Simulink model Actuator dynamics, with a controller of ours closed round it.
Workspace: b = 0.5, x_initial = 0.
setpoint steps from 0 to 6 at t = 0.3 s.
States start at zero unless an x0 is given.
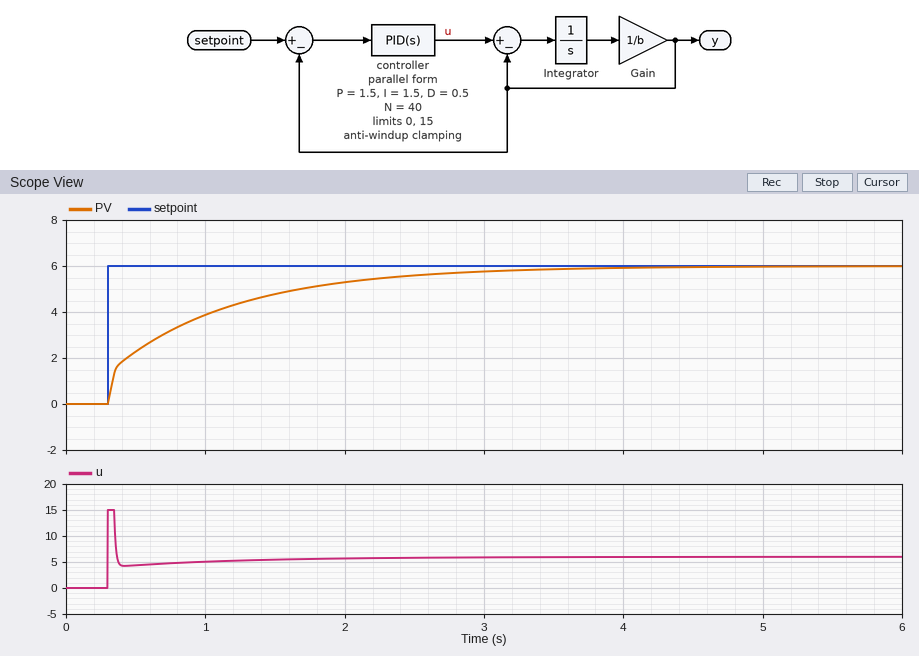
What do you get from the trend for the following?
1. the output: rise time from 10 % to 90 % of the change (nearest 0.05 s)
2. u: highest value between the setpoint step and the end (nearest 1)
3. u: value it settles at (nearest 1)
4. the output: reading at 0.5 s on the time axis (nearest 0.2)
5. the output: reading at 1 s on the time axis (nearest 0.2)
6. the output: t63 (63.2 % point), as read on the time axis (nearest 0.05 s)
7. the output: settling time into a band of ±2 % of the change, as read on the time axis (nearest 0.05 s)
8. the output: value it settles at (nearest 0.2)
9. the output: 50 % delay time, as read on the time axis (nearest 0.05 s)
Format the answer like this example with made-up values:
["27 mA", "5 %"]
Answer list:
["1.85 s", "15", "6", "2.2", "3.8", "0.95 s", "3.65 s", "6.0", "0.70 s"]
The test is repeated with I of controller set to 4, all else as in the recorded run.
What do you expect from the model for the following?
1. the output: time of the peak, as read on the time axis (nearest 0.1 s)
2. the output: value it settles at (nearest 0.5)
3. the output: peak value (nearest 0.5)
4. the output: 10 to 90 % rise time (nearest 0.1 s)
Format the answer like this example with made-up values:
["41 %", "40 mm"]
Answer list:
["2.0 s", "6.0", "6.5", "0.8 s"]
